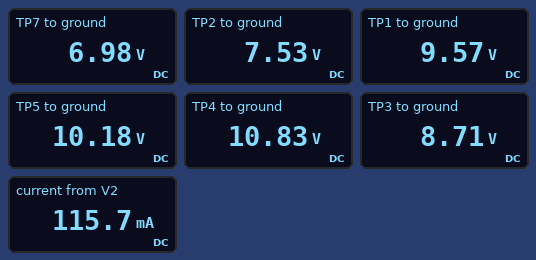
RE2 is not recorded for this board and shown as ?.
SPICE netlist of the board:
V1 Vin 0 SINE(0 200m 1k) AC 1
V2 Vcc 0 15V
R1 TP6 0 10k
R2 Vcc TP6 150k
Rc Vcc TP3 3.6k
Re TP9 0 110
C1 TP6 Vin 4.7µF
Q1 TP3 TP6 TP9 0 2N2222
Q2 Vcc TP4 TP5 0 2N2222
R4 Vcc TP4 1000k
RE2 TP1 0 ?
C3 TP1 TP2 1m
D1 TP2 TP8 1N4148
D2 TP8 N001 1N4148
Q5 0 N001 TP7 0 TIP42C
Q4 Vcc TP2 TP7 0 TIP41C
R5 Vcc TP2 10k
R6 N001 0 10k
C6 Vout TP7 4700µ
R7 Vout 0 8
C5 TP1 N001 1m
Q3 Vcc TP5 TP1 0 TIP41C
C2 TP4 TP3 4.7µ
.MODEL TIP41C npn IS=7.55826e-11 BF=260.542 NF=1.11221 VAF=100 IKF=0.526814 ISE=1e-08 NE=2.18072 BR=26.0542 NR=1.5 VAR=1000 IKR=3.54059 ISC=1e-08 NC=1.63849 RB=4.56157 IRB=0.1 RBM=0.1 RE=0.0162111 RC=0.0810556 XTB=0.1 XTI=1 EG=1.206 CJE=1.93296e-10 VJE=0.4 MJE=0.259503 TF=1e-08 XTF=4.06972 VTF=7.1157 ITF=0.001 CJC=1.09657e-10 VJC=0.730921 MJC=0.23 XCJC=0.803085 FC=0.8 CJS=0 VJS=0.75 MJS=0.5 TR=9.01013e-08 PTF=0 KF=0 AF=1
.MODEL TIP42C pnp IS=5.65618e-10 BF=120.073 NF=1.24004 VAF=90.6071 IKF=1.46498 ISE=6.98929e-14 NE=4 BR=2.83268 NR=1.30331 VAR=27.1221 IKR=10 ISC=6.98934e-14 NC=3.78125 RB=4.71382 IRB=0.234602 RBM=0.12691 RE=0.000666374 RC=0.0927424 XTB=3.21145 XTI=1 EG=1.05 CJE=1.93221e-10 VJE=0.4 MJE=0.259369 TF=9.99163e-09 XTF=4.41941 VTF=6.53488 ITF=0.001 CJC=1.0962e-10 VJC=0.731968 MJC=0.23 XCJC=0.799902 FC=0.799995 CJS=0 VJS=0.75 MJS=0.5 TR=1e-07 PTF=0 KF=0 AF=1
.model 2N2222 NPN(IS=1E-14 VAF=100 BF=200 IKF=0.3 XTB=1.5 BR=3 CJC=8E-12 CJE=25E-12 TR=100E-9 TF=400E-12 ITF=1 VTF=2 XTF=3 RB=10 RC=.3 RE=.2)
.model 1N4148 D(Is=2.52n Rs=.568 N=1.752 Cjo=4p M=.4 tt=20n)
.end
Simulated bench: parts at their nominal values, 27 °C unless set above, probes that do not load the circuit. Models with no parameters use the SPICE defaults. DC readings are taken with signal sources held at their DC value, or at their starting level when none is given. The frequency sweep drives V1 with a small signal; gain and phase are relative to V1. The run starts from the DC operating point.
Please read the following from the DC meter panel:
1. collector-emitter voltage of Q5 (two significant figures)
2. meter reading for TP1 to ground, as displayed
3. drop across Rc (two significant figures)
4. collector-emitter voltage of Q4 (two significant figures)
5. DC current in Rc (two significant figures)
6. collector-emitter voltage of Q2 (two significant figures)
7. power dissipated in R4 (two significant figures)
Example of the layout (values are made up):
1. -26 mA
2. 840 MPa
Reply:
1. -7.0 V
2. 9.57 V
3. 6.3 V
4. 8.0 V
5. 1.7 mA
6. 4.8 V
7. 17 µW
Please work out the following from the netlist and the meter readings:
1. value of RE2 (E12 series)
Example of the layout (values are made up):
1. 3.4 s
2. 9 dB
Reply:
1. 100 Ω
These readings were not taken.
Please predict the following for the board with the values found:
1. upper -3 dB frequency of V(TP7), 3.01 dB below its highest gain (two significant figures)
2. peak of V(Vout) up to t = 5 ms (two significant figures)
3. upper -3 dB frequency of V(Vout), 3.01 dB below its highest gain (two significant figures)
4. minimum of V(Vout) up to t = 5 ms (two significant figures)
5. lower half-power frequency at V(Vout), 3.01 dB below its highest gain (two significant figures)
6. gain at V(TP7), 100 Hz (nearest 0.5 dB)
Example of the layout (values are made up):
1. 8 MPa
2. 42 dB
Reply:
1. 1.7 MHz
2. 4.6 V
3. 1.7 MHz
4. -5.6 V
5. 910 kHz
6. 28.0 dB
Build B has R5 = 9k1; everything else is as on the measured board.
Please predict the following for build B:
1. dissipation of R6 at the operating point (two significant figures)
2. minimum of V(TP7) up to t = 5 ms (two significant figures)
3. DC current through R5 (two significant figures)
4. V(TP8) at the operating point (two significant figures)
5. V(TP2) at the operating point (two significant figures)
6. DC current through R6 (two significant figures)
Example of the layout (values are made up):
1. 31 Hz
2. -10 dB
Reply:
1. 4.6 mW
2. 1.7 V
3. 780 µA
4. 7.3 V
5. 7.9 V
6. 680 µA
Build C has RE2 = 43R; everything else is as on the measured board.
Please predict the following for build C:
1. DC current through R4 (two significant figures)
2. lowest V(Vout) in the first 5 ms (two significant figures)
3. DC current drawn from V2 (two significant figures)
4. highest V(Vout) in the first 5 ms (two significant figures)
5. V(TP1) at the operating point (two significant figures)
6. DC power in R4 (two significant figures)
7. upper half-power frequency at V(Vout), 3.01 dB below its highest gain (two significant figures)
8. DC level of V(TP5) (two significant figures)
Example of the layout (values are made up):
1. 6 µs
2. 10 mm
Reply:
1. 6.6 µA
2. -5.5 V
3. 190 mA
4. 4.9 V
5. 7.1 V
6. 43 µW
7. 1.9 MHz
8. 7.8 V
